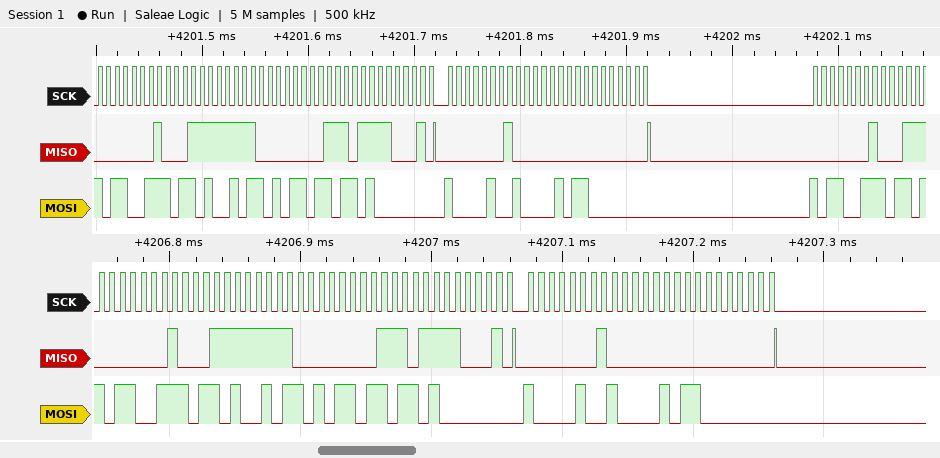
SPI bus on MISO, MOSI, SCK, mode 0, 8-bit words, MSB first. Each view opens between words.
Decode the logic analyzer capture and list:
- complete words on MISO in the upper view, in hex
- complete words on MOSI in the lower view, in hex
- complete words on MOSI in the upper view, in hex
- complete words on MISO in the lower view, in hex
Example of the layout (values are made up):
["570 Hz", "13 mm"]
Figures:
["01, 1F, E0, 1D, E2, 01, 00, 00, 01", "B3, B4, B5, B6, 80, 84, 85, 80", "B3, B4, B5, B6, 80, 84, 85, 80, B3", "01, 1F, E0, 1D, E2, 01, 00, 00"]
